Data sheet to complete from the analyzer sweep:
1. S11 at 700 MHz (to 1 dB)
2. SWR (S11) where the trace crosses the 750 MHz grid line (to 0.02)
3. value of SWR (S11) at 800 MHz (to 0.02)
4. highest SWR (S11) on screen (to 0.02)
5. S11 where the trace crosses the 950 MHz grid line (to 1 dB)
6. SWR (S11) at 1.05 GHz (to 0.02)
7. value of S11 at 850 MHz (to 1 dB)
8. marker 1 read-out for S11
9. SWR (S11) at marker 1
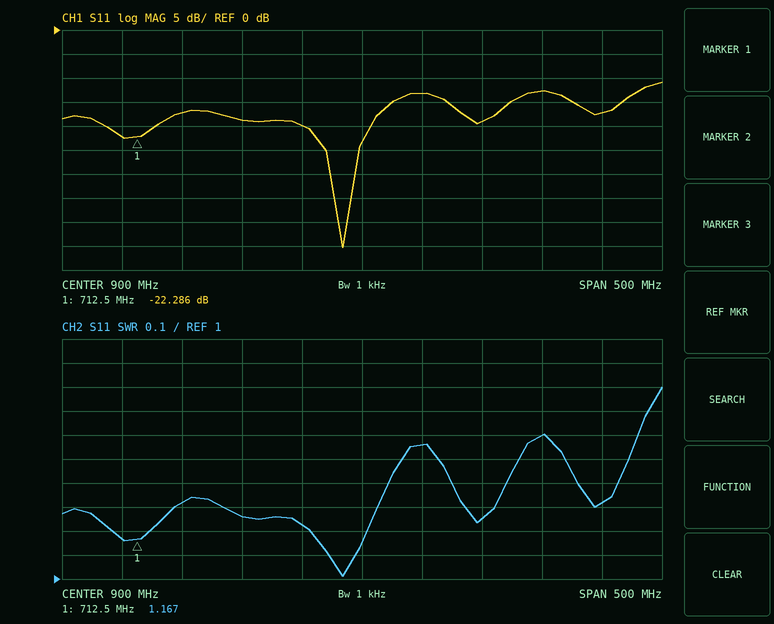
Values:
-22 dB
1.32
1.26
1.80
-13 dB
1.60
-20 dB
-22.286 dB
1.167
